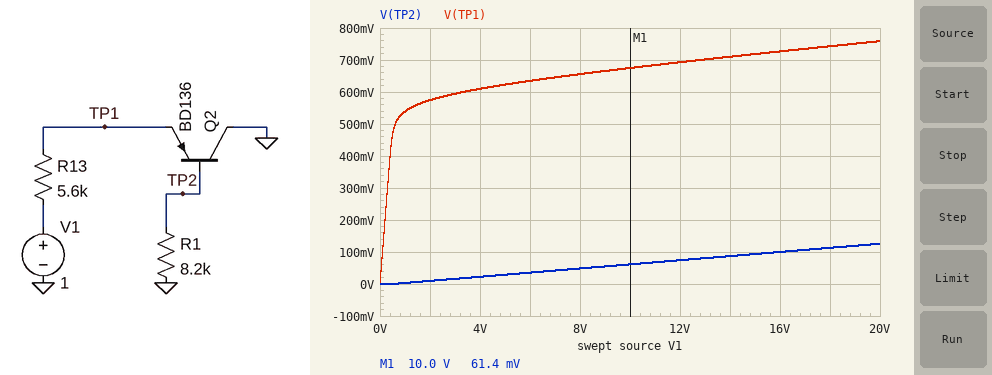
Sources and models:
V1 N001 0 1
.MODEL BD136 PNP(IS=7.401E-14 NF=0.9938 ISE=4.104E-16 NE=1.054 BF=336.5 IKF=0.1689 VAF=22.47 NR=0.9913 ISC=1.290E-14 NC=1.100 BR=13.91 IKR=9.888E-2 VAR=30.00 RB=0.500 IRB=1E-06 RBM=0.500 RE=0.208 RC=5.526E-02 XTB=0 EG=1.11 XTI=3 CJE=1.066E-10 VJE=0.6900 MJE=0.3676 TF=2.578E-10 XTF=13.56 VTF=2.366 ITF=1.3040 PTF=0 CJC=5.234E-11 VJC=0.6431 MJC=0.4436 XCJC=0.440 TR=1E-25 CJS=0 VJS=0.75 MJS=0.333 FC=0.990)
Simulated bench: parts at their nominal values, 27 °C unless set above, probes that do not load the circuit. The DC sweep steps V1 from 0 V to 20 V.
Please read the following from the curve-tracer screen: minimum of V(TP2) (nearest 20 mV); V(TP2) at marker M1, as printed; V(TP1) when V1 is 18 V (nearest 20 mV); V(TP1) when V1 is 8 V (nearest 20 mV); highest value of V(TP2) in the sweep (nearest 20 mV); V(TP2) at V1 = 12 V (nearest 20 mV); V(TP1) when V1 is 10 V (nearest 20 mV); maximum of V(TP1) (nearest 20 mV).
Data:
0 V
61.4 mV
740 mV
660 mV
120 mV
80 mV
680 mV
760 mV
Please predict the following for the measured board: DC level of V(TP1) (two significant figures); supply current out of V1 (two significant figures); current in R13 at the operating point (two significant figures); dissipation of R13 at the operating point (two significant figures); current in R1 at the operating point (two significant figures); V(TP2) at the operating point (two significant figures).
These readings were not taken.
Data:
540 mV
82 µA
82 µA
38 µW
390 nA
3.2 mV
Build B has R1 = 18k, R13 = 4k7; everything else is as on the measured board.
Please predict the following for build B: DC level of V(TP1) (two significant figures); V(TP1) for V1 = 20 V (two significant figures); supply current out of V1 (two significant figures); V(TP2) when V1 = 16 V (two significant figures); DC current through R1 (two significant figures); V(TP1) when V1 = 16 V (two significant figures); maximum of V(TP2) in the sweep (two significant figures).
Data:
550 mV
960 mV
96 µA
260 mV
450 nA
890 mV
320 mV
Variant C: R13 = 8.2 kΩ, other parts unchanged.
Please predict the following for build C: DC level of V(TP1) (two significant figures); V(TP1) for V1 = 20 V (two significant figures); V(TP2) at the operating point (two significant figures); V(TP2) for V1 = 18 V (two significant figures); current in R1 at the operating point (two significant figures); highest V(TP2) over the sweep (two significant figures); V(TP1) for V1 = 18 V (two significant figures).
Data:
530 mV
710 mV
2.2 mV
78 mV
270 nA
86 mV
700 mV
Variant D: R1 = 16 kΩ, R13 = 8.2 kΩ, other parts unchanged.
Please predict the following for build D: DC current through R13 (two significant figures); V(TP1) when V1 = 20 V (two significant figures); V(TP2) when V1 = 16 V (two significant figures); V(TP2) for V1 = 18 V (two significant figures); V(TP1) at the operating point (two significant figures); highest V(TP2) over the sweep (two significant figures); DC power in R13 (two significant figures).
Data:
57 µA
790 mV
130 mV
150 mV
530 mV
170 mV
27 µW
